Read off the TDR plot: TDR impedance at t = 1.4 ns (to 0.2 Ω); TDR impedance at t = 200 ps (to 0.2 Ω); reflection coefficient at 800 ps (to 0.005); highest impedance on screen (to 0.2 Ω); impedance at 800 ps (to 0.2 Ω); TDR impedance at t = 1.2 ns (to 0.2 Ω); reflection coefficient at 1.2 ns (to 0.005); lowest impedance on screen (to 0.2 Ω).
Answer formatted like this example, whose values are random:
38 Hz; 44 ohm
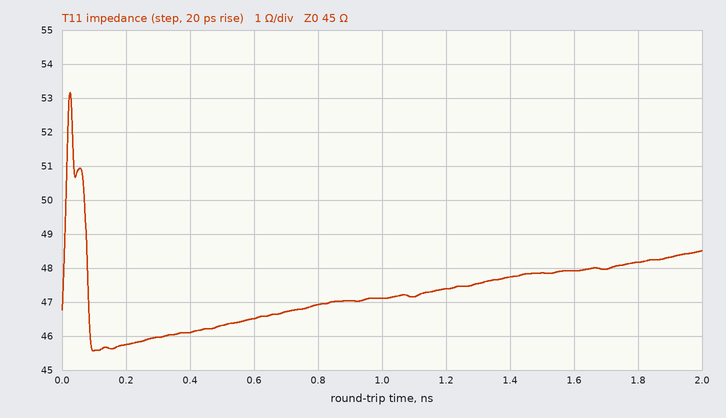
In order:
47.8 Ω; 45.8 Ω; +0.020; 53.2 Ω; 47.0 Ω; 47.4 Ω; +0.025; 45.6 Ω
